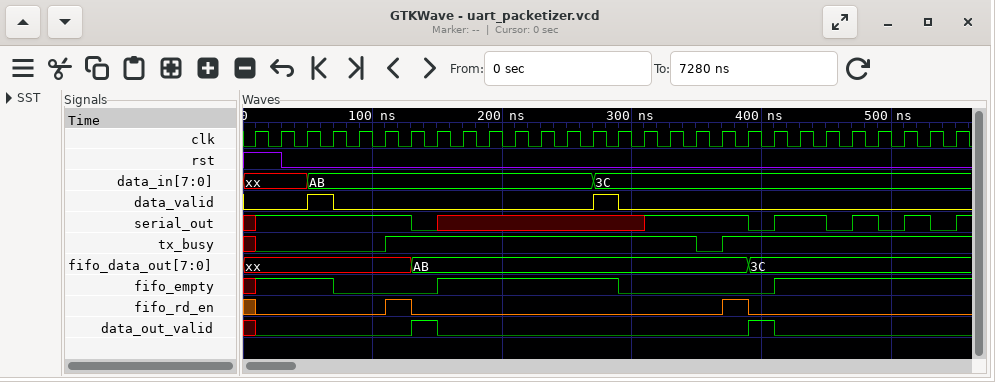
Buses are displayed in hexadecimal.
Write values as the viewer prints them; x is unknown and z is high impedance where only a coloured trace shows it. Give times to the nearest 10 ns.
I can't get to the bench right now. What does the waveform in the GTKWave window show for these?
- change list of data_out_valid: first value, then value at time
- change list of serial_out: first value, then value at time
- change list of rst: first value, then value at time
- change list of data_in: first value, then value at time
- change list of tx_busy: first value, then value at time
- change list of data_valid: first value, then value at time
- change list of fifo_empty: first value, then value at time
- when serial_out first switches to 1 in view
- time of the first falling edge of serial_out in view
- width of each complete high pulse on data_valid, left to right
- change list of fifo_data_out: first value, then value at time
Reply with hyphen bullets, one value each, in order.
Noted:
- x, 0 at 10 ns, 1 at 130 ns, 0 at 150 ns, 1 at 390 ns, 0 at 410 ns
- x, 1 at 10 ns, 0 at 130 ns, x at 150 ns, 1 at 310 ns, 0 at 390 ns, 1 at 410 ns, 0 at 450 ns, 1 at 470 ns, 0 at 490 ns, 1 at 510 ns, 0 at 530 ns, 1 at 550 ns
- 1, 0 at 30 ns
- xx, AB at 50 ns, 3C at 270 ns
- x, 0 at 10 ns, 1 at 110 ns, 0 at 350 ns, 1 at 370 ns
- 0, 1 at 50 ns, 0 at 70 ns, 1 at 270 ns, 0 at 290 ns
- x, 1 at 10 ns, 0 at 70 ns, 1 at 150 ns, 0 at 290 ns, 1 at 410 ns
- 10 ns
- 130 ns
- 20 ns, 20 ns
- xx, AB at 130 ns, 3C at 390 ns
